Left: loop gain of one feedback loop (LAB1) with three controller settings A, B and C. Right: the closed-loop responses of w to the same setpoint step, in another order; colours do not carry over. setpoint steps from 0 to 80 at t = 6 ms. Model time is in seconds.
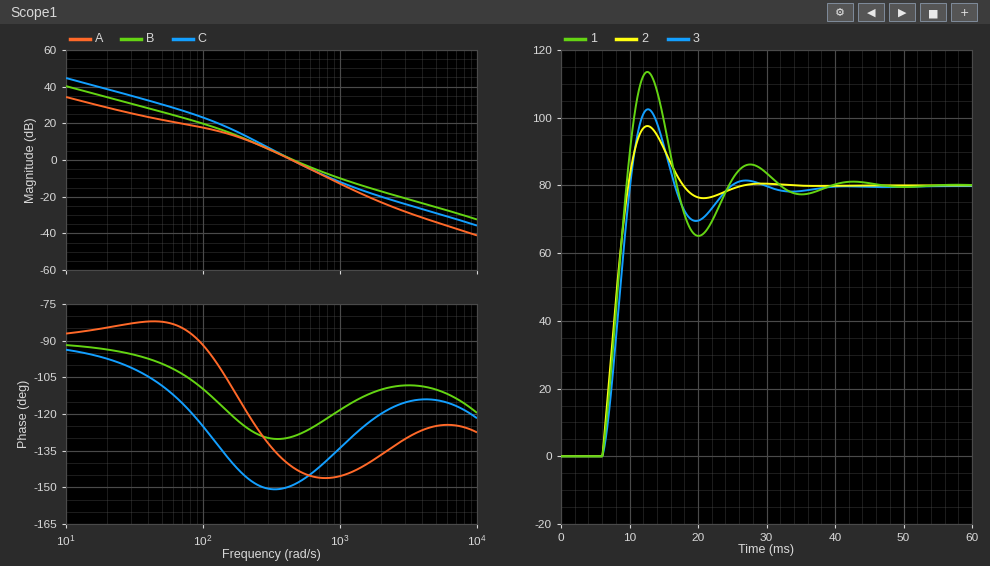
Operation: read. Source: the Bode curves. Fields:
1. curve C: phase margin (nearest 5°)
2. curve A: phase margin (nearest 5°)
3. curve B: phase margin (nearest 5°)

30°
40°
50°
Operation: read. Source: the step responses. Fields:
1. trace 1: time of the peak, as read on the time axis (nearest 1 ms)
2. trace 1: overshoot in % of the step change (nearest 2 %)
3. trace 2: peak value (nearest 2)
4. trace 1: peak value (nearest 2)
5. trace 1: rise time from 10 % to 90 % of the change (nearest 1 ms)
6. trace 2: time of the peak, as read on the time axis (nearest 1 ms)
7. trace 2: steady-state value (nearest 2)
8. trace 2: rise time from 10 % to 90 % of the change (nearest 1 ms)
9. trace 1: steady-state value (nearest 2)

13 ms
42 %
98
114
3 ms
13 ms
80
3 ms
80
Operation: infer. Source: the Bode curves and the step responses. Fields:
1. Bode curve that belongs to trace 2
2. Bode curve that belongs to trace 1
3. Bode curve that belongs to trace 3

B
C
A
